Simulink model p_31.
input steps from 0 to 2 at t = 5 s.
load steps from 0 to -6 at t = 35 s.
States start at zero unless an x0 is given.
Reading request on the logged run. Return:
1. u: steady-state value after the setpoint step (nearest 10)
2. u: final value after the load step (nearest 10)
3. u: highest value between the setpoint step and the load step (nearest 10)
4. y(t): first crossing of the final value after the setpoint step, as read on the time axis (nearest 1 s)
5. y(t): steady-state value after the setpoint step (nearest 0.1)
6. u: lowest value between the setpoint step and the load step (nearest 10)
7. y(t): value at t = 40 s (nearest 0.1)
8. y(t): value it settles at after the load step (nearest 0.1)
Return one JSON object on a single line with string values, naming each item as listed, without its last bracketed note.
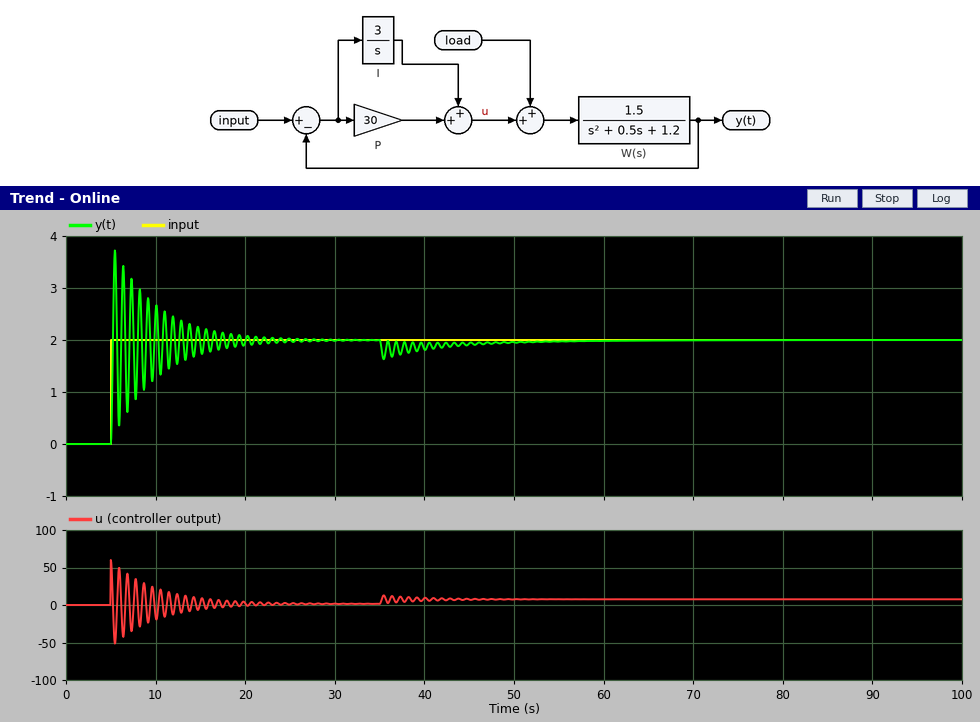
{"u: steady-state value after the setpoint step": "0", "u: final value after the load step": "10", "u: highest value between the setpoint step and the load step": "60", "y(t): first crossing of the final value after the setpoint step, as read on the time axis": "5 s", "y(t): steady-state value after the setpoint step": "2.0", "u: lowest value between the setpoint step and the load step": "-50", "y(t): value at t = 40 s": "1.8", "y(t): value it settles at after the load step": "2.0"}
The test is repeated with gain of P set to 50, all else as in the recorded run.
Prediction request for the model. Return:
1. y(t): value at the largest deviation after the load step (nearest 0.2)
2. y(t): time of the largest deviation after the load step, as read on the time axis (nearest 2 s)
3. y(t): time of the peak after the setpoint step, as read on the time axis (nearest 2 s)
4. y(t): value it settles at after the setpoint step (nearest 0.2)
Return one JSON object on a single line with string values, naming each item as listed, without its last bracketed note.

{"y(t): value at the largest deviation after the load step": "1.8", "y(t): time of the largest deviation after the load step, as read on the time axis": "36 s", "y(t): time of the peak after the setpoint step, as read on the time axis": "6 s", "y(t): value it settles at after the setpoint step": "2.0"}
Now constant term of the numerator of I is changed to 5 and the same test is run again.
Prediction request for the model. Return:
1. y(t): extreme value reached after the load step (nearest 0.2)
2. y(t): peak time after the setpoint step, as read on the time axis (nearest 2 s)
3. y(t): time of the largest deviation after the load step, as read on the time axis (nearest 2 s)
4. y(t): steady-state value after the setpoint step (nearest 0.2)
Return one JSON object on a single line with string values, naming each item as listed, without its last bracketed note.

{"y(t): extreme value reached after the load step": "1.6", "y(t): peak time after the setpoint step, as read on the time axis": "6 s", "y(t): time of the largest deviation after the load step, as read on the time axis": "36 s", "y(t): steady-state value after the setpoint step": "2.0"}
